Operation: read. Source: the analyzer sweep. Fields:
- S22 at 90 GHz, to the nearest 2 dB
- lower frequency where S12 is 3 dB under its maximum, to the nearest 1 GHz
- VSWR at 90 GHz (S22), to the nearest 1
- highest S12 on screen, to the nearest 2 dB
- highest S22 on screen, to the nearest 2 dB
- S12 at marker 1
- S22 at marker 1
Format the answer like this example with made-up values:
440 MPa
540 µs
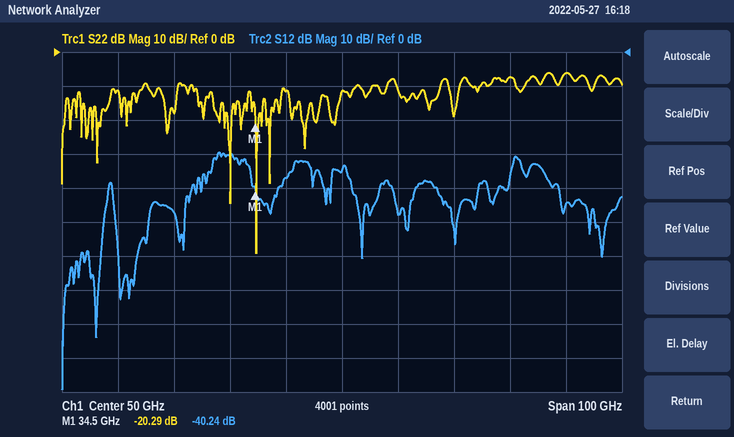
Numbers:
-6 dB
27 GHz
3
-30 dB
-6 dB
-40.24 dB
-20.29 dB
